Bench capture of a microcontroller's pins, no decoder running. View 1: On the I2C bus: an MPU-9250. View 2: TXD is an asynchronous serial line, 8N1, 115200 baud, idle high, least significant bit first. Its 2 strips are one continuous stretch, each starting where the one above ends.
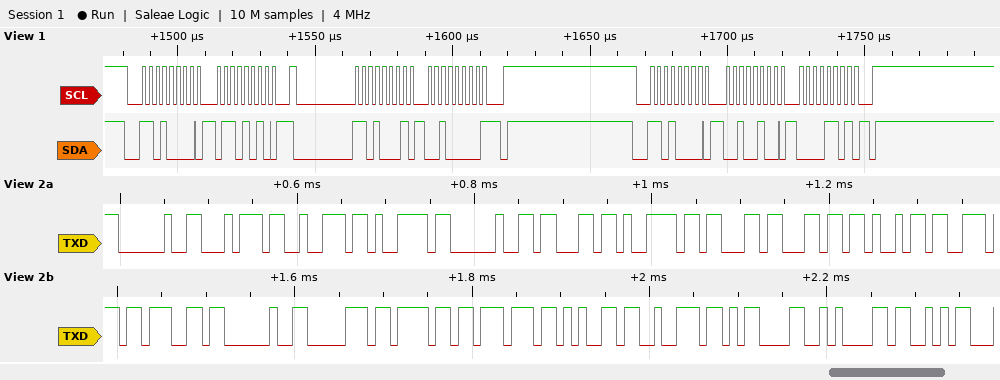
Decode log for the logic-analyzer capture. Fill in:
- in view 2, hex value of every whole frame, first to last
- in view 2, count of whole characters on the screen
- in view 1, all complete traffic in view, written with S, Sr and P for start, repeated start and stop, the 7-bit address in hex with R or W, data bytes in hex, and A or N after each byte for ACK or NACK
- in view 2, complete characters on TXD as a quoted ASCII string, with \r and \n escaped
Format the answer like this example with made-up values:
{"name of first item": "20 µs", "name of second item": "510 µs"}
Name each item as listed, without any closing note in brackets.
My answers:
{"in view 2, hex value of every whole frame, first to last": "20 74 72 79 20 63 79 63 6C 69 6E 67 20 70 6F 77 65 72 0D 0A 53", "in view 2, count of whole characters on the screen": "21", "in view 1, all complete traffic in view, written with S, Sr and P for start, repeated start and stop, the 7-bit address in hex with R or W, data bytes in hex, and A or N after each byte for ACK or NACK": "S 68W A 6A A Sr 68R A 20 N P S 68W A 24 A 0D A P", "in view 2, complete characters on TXD as a quoted ASCII string, with \\r and \\n escaped": "\" try cycling power\\r\\nS\""}
